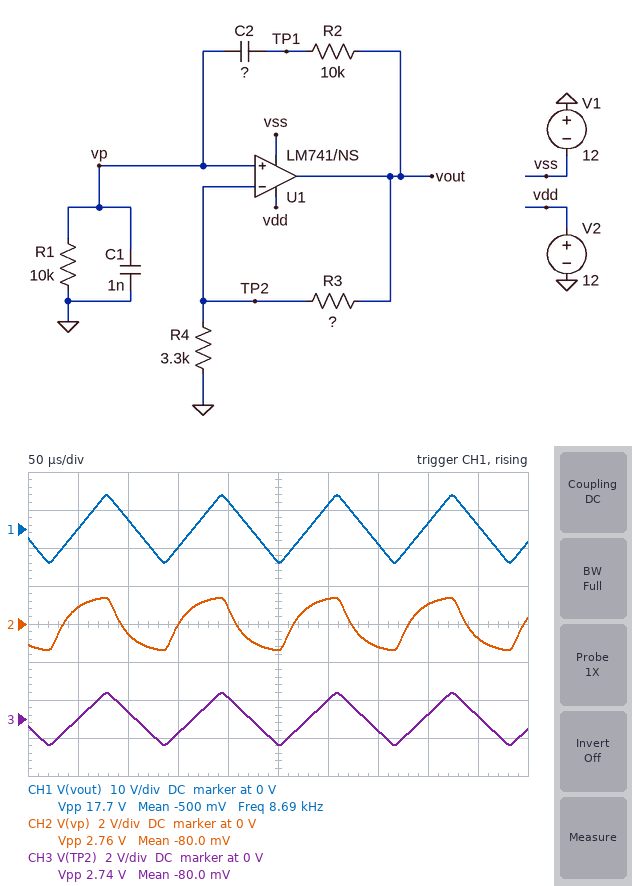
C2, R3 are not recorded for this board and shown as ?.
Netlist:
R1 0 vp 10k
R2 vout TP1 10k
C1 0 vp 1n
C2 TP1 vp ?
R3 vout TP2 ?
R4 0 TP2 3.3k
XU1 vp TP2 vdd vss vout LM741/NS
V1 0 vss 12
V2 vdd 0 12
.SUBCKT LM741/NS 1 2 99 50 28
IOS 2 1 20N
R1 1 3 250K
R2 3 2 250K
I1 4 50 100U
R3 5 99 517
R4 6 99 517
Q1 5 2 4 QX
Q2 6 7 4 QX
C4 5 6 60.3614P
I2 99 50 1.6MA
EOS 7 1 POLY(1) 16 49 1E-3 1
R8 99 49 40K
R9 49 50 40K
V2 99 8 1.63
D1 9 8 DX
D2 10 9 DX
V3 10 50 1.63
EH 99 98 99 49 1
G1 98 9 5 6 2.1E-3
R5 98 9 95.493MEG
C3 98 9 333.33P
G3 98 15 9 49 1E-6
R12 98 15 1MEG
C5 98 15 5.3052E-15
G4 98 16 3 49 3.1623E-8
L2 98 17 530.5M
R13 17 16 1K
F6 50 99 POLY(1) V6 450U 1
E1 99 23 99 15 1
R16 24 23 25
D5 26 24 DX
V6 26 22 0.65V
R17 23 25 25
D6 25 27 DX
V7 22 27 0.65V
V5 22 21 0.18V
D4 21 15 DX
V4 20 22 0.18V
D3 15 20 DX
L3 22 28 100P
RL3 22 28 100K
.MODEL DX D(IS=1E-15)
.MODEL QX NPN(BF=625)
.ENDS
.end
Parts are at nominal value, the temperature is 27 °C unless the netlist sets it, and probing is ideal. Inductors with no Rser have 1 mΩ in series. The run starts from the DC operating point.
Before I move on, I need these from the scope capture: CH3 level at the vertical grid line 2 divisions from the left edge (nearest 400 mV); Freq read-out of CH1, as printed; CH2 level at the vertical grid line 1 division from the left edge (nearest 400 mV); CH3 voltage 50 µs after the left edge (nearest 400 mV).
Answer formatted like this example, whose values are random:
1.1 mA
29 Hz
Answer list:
400 mV
8.69 kHz
800 mV
0 V
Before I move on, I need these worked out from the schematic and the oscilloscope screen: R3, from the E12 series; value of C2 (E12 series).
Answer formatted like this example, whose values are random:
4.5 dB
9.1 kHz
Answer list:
18 kΩ
470 pF
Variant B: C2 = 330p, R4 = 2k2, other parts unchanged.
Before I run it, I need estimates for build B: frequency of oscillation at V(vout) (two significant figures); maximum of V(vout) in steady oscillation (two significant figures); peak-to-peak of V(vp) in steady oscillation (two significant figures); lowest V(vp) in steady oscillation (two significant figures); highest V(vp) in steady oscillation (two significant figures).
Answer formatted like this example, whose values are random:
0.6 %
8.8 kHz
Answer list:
8.5 kHz
9.1 V
2.0 V
-1.0 V
1.0 V
